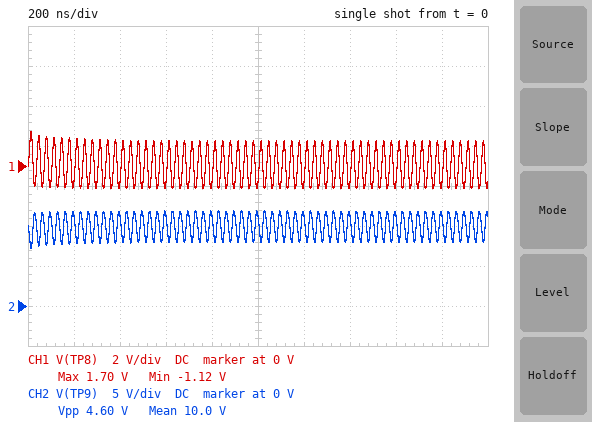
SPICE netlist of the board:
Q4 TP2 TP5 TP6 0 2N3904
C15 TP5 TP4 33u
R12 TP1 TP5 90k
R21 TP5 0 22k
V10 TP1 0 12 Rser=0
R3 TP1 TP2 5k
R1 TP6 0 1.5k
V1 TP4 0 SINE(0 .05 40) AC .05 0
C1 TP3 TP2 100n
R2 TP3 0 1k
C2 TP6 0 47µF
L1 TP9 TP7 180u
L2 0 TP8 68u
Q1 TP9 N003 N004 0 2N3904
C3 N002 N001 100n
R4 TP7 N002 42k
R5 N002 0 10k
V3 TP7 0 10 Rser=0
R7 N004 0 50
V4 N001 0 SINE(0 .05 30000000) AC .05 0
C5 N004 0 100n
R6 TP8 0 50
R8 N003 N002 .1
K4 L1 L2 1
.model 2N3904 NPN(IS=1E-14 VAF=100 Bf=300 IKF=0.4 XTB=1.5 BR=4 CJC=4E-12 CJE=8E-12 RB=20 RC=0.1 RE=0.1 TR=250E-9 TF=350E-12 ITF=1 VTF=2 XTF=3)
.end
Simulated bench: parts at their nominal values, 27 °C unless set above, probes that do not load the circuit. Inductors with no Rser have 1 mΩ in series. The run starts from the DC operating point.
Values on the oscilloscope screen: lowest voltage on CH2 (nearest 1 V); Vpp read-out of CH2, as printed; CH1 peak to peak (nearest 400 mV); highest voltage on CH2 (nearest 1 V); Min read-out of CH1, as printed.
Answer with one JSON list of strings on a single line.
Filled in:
["7 V", "4.60 V", "2.8 V", "12 V", "-1.12 V"]
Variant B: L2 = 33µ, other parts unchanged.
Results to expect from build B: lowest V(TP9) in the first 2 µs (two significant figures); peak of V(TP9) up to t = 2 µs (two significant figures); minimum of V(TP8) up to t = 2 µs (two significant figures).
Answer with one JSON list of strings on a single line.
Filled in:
["5.5 V", "13 V", "-1.4 V"]
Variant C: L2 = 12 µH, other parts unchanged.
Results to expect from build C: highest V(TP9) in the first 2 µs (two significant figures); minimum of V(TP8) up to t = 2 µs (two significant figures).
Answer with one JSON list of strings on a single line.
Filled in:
["16 V", "-1.5 V"]
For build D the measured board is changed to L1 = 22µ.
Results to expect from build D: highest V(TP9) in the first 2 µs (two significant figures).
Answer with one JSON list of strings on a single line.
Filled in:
["10 V"]
